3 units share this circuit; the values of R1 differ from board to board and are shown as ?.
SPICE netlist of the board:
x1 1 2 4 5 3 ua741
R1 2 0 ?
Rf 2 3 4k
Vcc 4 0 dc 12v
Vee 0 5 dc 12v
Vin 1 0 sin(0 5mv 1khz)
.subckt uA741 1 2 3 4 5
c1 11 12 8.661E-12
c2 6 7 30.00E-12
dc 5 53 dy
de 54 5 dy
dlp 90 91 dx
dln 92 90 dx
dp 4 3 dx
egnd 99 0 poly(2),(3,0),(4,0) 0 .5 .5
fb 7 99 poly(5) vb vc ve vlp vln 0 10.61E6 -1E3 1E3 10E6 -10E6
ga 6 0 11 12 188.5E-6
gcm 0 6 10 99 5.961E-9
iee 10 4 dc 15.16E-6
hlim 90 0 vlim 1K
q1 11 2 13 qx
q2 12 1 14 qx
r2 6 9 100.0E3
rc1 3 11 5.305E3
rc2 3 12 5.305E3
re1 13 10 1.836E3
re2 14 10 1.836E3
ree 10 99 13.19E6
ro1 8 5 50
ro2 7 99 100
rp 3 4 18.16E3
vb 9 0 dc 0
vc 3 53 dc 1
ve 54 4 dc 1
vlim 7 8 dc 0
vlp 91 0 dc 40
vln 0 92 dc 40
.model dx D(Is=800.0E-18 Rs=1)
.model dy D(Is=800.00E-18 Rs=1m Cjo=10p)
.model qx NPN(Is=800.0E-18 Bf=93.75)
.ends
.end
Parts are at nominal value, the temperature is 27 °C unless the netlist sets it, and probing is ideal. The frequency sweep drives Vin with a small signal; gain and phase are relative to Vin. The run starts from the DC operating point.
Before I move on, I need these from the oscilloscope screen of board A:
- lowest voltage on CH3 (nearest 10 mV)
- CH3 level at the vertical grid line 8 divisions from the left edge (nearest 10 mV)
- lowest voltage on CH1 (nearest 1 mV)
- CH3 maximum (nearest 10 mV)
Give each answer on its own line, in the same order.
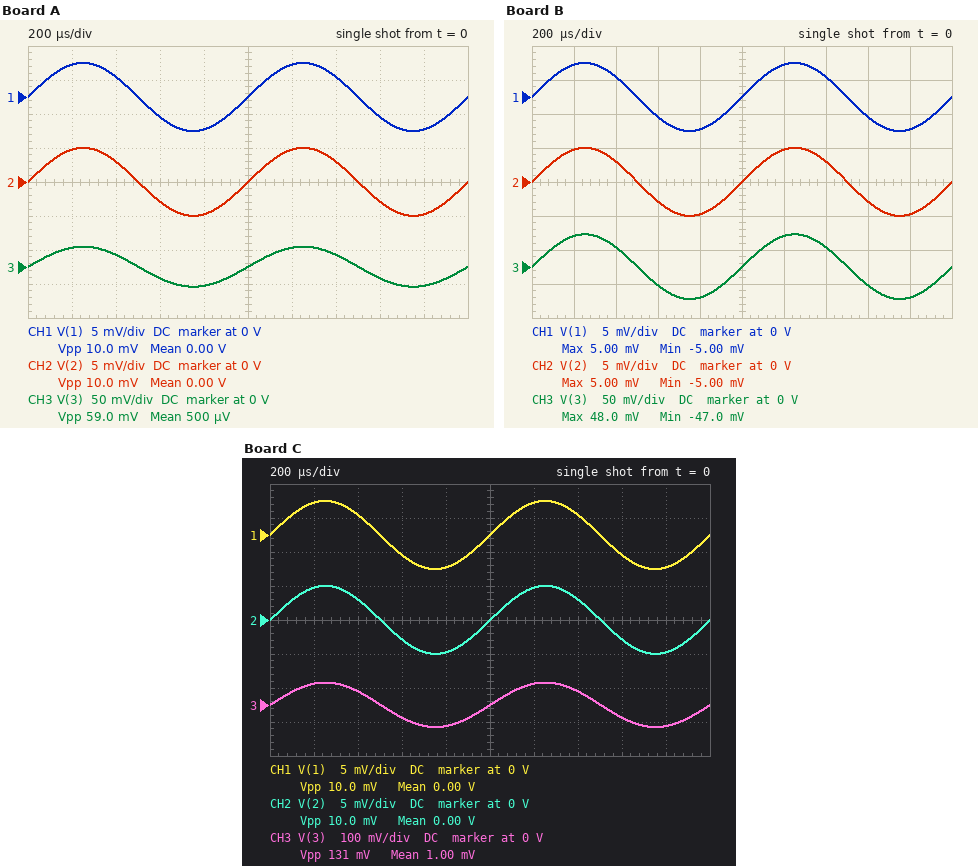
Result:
-30 mV
-20 mV
-5 mV
30 mV
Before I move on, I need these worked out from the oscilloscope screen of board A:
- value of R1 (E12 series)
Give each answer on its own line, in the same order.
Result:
820 Ω
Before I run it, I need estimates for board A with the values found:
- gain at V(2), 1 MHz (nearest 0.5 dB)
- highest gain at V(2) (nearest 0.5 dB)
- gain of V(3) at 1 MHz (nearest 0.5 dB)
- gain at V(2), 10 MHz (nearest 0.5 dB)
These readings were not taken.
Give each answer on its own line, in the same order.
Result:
-16.0 dB
0 dB
-1.0 dB
-53.0 dB
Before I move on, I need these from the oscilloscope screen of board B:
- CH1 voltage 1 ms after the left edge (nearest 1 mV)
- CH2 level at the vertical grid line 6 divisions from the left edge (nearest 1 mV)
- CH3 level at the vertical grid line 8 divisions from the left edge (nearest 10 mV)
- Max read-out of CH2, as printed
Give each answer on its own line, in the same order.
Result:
0 V
5 mV
-30 mV
5.00 mV
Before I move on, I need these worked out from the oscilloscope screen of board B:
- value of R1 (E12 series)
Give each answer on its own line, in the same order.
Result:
470 Ω
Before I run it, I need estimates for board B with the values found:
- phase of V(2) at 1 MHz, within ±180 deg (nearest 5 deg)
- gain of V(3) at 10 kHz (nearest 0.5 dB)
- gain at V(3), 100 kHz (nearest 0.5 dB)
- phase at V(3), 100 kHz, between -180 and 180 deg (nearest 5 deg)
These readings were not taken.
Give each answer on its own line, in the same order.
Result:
-115 deg
19.5 dB
17.0 dB
-45 deg
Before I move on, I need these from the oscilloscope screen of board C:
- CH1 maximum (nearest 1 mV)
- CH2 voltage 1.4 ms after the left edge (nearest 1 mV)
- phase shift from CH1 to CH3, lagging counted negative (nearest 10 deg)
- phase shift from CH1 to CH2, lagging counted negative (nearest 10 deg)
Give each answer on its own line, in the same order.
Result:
5 mV
3 mV
0 deg
0 deg
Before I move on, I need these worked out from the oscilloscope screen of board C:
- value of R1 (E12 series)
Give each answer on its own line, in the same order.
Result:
330 Ω
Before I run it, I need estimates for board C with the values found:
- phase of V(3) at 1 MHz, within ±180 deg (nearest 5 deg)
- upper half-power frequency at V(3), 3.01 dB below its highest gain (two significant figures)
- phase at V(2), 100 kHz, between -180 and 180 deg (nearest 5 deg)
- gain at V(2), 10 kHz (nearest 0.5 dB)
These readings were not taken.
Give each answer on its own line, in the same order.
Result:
-115 deg
79 kHz
-55 deg
0 dB
